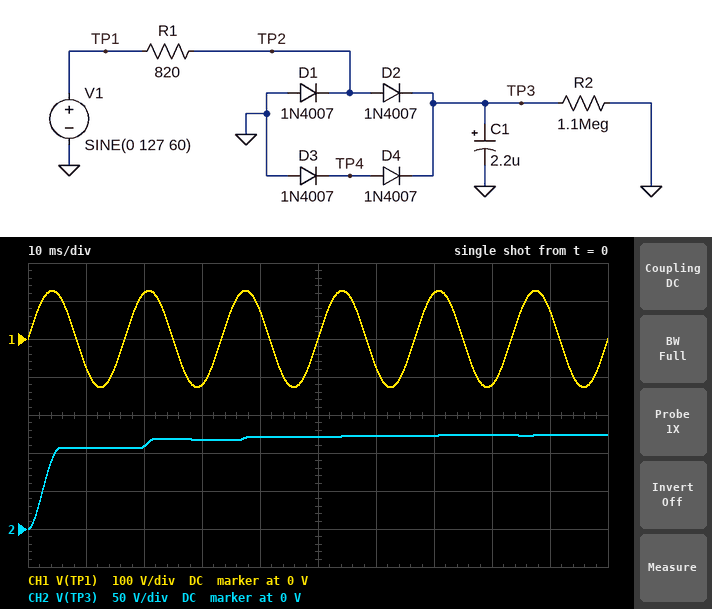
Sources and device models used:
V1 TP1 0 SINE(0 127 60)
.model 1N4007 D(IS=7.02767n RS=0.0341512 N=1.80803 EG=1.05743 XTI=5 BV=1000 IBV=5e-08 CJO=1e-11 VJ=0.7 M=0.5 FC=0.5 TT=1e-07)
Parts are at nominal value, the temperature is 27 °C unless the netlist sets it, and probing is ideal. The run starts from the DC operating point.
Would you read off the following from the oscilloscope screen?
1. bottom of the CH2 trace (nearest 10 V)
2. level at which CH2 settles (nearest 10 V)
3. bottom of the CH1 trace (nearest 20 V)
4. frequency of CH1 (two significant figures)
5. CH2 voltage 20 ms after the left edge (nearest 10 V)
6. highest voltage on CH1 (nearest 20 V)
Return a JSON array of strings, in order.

["0 V", "120 V", "-120 V", "60 Hz", "110 V", "120 V"]
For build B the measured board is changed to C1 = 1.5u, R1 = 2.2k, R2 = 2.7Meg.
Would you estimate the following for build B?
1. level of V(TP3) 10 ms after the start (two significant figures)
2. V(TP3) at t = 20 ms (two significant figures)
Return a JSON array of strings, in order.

["88 V", "94 V"]
